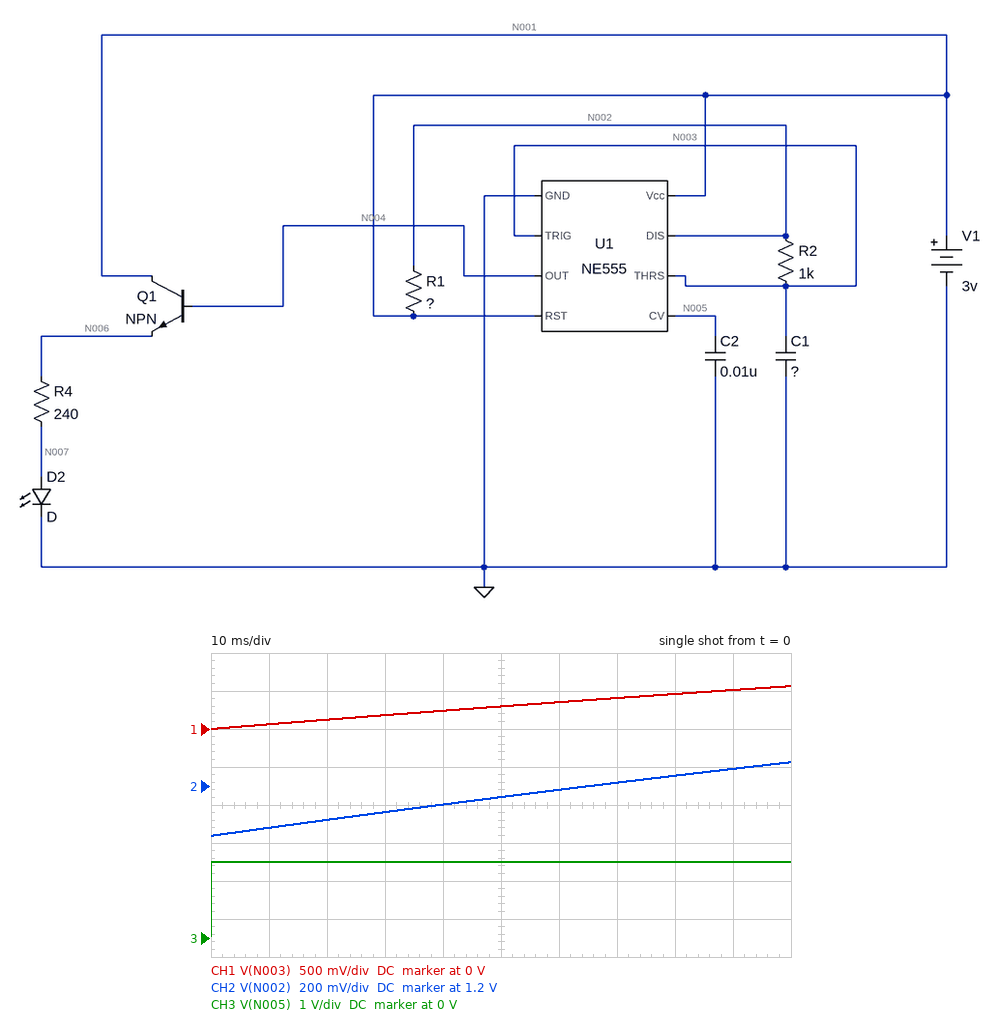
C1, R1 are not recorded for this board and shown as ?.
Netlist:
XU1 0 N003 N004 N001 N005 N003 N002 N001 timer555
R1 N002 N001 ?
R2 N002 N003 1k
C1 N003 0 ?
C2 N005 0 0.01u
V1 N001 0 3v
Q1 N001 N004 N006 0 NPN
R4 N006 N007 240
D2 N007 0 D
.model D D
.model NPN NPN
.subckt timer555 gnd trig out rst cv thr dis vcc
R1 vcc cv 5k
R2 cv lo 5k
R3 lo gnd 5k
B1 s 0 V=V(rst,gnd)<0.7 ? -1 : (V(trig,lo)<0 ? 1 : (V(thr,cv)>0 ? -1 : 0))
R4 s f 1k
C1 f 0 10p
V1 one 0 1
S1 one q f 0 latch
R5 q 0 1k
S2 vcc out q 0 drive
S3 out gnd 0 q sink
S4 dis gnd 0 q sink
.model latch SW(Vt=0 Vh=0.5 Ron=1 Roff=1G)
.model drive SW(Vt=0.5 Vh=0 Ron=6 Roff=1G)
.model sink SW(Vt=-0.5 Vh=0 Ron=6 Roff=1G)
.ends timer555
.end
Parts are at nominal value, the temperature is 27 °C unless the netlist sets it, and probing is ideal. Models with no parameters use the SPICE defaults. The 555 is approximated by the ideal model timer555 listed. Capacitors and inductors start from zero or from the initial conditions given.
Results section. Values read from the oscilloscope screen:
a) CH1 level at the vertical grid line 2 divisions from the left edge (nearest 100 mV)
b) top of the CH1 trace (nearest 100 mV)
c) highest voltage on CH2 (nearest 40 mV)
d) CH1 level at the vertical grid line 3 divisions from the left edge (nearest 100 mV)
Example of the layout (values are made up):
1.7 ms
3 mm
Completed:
100 mV
600 mV
1.32 V
200 mV
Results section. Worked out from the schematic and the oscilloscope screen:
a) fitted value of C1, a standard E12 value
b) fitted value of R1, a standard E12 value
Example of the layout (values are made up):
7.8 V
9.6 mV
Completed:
150 µF
2.2 kΩ
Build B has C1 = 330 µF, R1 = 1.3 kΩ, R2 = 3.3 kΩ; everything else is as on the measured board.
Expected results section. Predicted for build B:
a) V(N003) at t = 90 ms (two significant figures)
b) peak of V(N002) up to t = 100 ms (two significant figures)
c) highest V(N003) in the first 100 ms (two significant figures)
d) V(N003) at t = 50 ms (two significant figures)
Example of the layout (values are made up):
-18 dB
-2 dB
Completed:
170 mV
2.2 V
190 mV
97 mV
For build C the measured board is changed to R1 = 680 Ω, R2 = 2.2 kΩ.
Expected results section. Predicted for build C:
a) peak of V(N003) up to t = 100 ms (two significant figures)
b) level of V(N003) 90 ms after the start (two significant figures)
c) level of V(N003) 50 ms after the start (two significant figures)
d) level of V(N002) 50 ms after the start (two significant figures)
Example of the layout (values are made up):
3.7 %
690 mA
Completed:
620 mV
560 mV
330 mV
2.4 V
